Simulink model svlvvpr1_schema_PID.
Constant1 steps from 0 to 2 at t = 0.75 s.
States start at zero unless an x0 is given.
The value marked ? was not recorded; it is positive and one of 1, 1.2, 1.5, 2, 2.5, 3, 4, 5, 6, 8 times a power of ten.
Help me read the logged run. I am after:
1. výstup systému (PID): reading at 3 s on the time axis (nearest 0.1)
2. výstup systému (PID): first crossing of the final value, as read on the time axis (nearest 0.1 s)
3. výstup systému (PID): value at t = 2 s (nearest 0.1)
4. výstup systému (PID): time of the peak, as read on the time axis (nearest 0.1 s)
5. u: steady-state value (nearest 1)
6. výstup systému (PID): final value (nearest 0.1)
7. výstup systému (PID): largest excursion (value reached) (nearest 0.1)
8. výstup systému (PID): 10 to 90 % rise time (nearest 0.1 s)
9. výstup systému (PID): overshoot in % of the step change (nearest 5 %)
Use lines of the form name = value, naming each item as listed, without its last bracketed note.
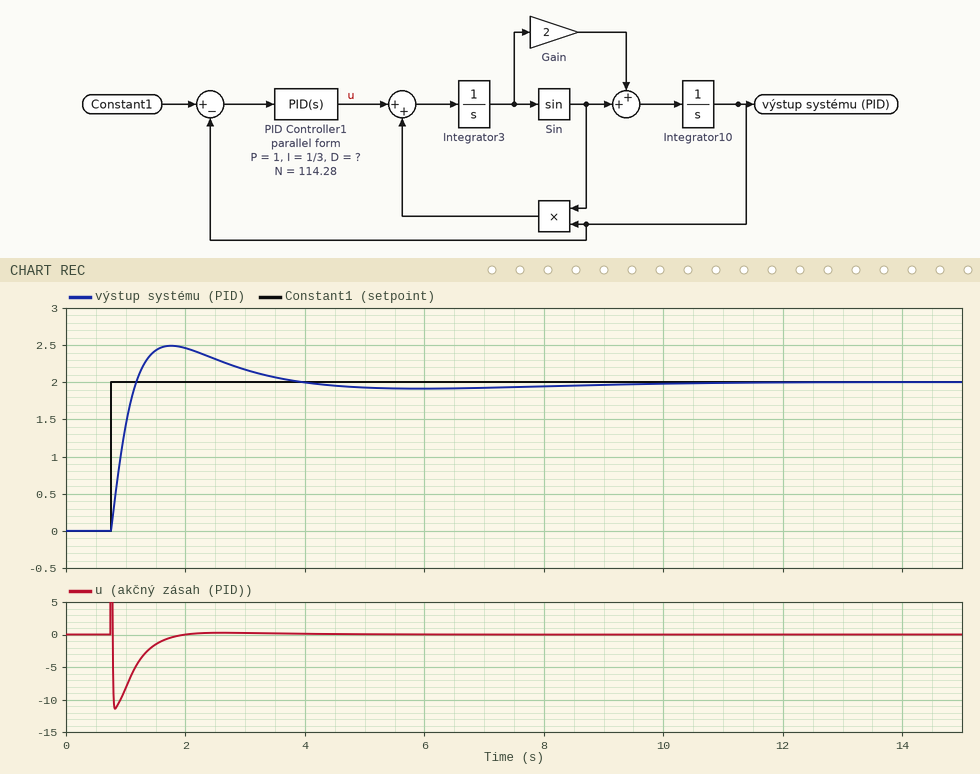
výstup systému (PID): reading at 3 s on the time axis = 2.2
výstup systému (PID): first crossing of the final value, as read on the time axis = 1.2 s
výstup systému (PID): value at t = 2 s = 2.5
výstup systému (PID): time of the peak, as read on the time axis = 1.8 s
u: steady-state value = 0
výstup systému (PID): final value = 2.0
výstup systému (PID): largest excursion (value reached) = 2.5
výstup systému (PID): 10 to 90 % rise time = 0.3 s
výstup systému (PID): overshoot in % of the step change = 25 %
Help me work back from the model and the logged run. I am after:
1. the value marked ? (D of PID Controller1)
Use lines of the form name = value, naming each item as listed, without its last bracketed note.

the value marked ? = 2
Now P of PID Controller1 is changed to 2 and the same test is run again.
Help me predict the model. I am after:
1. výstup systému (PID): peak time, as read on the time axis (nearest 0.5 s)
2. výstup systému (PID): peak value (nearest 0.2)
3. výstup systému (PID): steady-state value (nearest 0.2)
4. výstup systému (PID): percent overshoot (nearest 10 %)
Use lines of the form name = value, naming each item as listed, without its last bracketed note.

výstup systému (PID): peak time, as read on the time axis = 1.5 s
výstup systému (PID): peak value = 2.6
výstup systému (PID): steady-state value = 2.0
výstup systému (PID): percent overshoot = 30 %
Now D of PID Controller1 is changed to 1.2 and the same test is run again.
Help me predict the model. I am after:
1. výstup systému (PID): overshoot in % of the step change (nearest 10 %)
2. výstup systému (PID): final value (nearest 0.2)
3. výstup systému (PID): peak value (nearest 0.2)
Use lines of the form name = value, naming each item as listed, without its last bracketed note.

výstup systému (PID): overshoot in % of the step change = 60 %
výstup systému (PID): final value = 2.0
výstup systému (PID): peak value = 3.2
